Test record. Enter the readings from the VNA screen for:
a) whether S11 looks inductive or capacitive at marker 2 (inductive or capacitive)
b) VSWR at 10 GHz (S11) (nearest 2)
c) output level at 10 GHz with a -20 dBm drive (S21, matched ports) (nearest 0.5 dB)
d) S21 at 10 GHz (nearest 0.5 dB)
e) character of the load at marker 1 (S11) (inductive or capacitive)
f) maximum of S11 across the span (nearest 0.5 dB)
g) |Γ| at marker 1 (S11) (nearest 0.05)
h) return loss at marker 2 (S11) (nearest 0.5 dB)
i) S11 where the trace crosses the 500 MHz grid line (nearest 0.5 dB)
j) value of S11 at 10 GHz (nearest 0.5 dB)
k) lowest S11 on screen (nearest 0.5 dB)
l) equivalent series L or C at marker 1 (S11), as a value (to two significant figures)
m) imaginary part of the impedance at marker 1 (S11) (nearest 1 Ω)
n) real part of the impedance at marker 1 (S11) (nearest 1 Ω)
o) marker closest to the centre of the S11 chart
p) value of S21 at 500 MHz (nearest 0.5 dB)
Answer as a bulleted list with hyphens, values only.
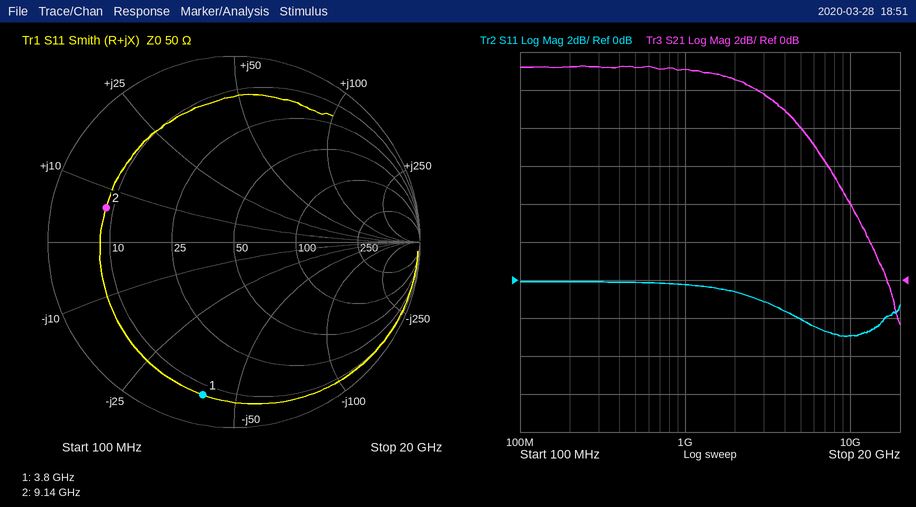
- inductive
- 6
- -16.0 dBm
- 4.0 dB
- capacitive
- 0.0 dB
- 0.85
- 3.0 dB
- 0.0 dB
- -3.0 dB
- -3.0 dB
- 1.0 pF
- -40 Ω
- 7 Ω
- marker 2
- 11.0 dB
